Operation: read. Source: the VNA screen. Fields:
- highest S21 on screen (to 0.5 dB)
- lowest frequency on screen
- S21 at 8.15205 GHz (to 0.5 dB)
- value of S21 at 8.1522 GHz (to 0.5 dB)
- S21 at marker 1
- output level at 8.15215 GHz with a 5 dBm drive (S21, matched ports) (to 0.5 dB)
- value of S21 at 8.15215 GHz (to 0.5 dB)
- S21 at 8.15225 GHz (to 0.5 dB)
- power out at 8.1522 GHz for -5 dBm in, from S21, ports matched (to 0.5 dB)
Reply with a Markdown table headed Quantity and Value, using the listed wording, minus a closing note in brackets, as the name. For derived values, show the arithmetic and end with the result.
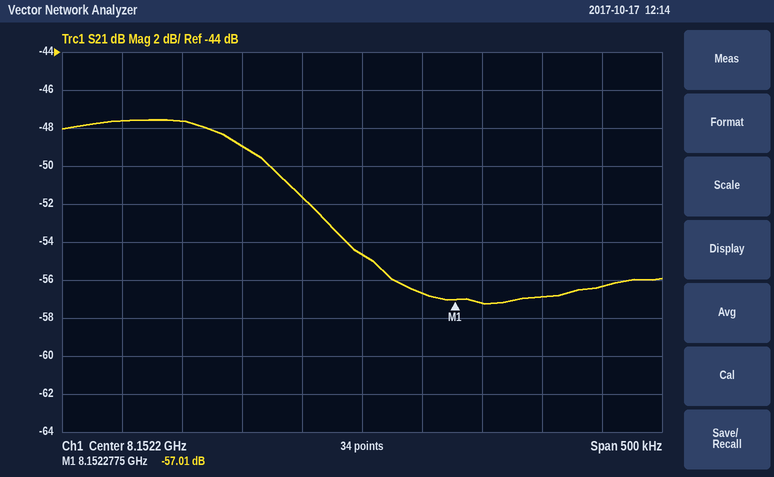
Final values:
| Quantity | Value |
|---|---|
| highest S21 on screen | -47.5 dB |
| lowest frequency on screen | 8.15195 GHz |
| S21 at 8.15205 GHz | -47.5 dB |
| value of S21 at 8.1522 GHz | -54.5 dB |
| S21 at marker 1 | -57.01 dB |
| output level at 8.15215 GHz with a 5 dBm drive (S21, matched ports) | 5 dBm + (-51.5 dB) = -46.5 dBm |
| value of S21 at 8.15215 GHz | -51.5 dB |
| S21 at 8.15225 GHz | -56.5 dB |
| power out at 8.1522 GHz for -5 dBm in, from S21, ports matched | -5 dBm + (-54.5 dB) = -59.5 dBm |
